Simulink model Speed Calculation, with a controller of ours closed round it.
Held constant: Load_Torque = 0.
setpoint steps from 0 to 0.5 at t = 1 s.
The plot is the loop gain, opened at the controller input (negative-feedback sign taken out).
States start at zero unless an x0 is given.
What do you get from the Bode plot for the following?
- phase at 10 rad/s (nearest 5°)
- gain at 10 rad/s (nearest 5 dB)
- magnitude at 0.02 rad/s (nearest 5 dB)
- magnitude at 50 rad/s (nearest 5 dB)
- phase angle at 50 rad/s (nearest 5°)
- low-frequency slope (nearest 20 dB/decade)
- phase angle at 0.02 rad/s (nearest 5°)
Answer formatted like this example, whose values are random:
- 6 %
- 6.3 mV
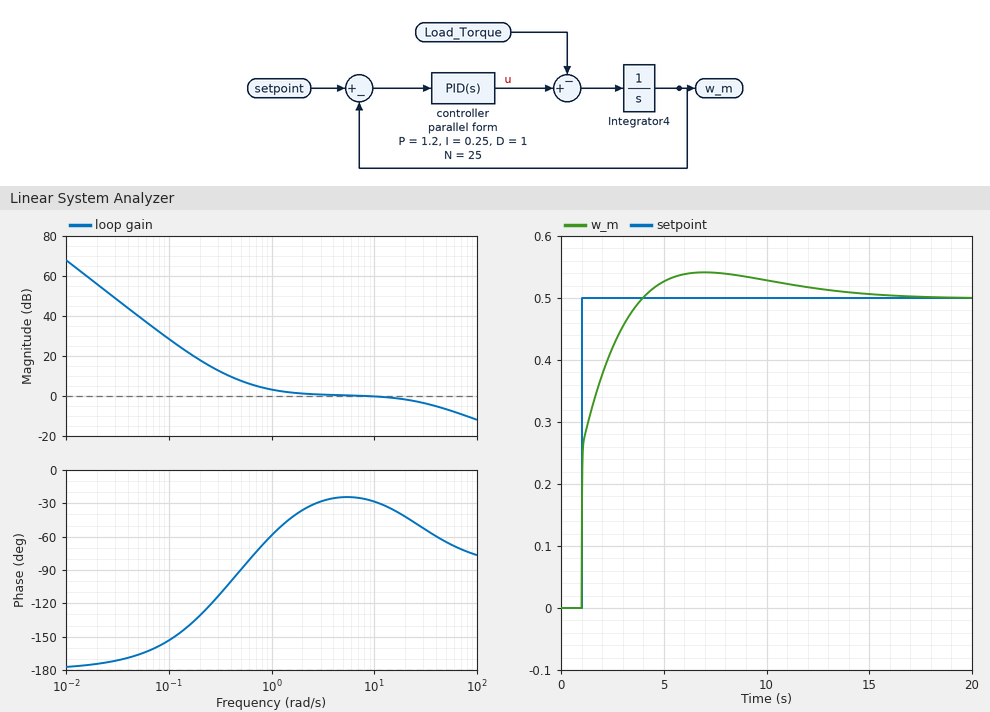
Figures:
- -30°
- 0 dB
- 55 dB
- -5 dB
- -65°
- -40 dB/decade
- -175°
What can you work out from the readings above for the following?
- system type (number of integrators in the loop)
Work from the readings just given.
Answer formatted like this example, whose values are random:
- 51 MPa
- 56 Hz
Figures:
- 2
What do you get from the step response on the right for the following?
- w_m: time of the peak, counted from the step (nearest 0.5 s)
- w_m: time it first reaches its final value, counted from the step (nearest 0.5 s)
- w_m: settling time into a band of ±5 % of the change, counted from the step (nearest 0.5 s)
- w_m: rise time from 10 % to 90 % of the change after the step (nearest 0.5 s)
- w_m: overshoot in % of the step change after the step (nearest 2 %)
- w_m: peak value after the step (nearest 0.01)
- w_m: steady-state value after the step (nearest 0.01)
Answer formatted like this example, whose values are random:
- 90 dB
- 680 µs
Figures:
- 6.0 s
- 3.0 s
- 9.5 s
- 2.0 s
- 8 %
- 0.54
- 0.50
